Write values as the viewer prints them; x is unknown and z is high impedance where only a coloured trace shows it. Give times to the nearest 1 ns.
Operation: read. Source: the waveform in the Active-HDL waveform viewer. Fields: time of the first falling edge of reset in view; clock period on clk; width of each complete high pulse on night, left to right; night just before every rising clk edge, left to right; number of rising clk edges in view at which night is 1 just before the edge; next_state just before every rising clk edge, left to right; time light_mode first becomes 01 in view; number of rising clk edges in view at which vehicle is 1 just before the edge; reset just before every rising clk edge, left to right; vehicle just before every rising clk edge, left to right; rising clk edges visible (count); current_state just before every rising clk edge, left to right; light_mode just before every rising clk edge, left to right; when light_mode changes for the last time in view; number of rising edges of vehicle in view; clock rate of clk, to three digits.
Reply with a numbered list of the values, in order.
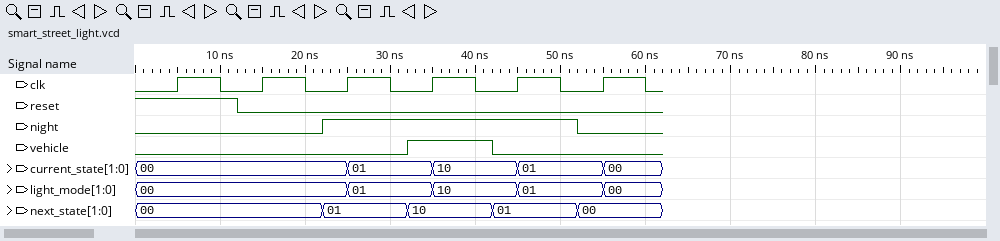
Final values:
1. 12 ns
2. 10 ns
3. 30 ns
4. 0 0 1 1 1 0
5. 3
6. 00, 00, 01, 10, 01, 00
7. 25 ns
8. 1
9. 1 0 0 0 0 0
10. 0 0 0 1 0 0
11. 6
12. 00, 00, 00, 01, 10, 01
13. 00, 00, 00, 01, 10, 01
14. 55 ns
15. 1
16. 100 MHz
